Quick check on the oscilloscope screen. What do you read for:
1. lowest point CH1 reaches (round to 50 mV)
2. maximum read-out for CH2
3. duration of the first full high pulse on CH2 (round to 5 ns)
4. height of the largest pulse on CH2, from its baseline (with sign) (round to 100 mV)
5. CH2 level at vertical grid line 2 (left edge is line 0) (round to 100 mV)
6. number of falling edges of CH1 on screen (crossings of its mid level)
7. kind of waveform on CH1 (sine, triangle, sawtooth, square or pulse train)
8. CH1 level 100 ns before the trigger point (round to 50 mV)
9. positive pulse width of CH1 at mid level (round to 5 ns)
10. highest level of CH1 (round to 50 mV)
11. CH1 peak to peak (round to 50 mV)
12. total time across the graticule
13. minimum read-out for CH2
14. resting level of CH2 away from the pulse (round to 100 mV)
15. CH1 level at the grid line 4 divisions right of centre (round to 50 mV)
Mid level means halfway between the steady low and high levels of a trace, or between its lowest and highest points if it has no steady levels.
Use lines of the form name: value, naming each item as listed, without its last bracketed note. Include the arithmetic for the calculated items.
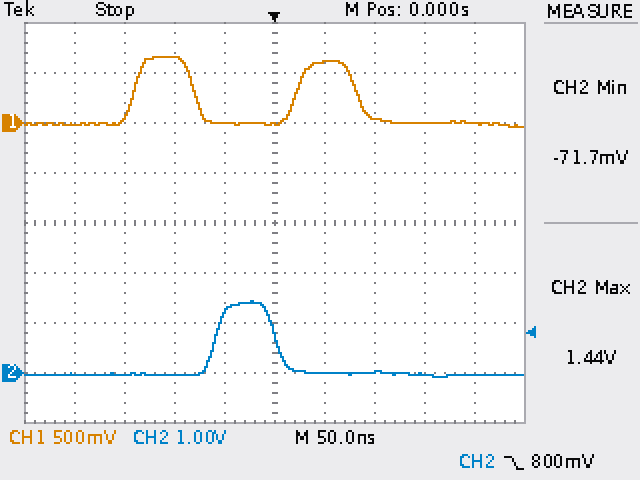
lowest point CH1 reaches: -50 mV
maximum read-out for CH2: 1.44 V
duration of the first full high pulse on CH2: 60 ns
height of the largest pulse on CH2, from its baseline (with sign): +1.5 V
CH2 level at vertical grid line 2 (left edge is line 0): 0.0 V
number of falling edges of CH1 on screen: 2
kind of waveform on CH1: pulse train
CH1 level 100 ns before the trigger point: 650 mV
positive pulse width of CH1 at mid level: 60 ns
highest level of CH1: 650 mV
CH1 peak to peak: 650 mV − (-50 mV) = 700 mV
total time across the graticule: 500 ns
minimum read-out for CH2: -71.7 mV
resting level of CH2 away from the pulse: 0.0 V
CH1 level at the grid line 4 divisions right of centre: 0 mV
